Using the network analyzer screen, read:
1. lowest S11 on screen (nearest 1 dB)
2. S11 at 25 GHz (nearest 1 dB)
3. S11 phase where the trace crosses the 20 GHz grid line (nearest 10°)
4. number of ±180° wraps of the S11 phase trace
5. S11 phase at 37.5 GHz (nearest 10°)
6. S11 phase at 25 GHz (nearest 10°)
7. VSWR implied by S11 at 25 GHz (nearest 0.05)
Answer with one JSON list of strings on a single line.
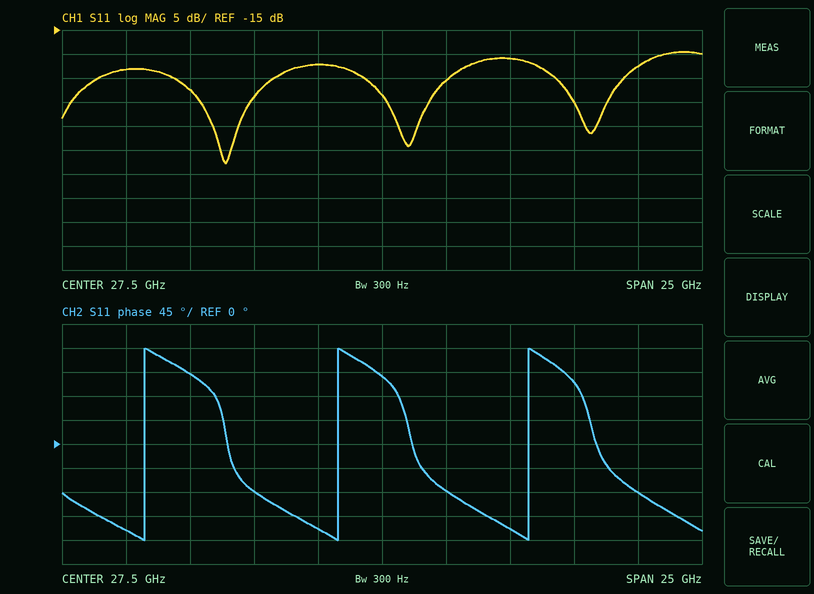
["-43 dB", "-22 dB", "130°", "3", "-90°", "-160°", "1.15"]
